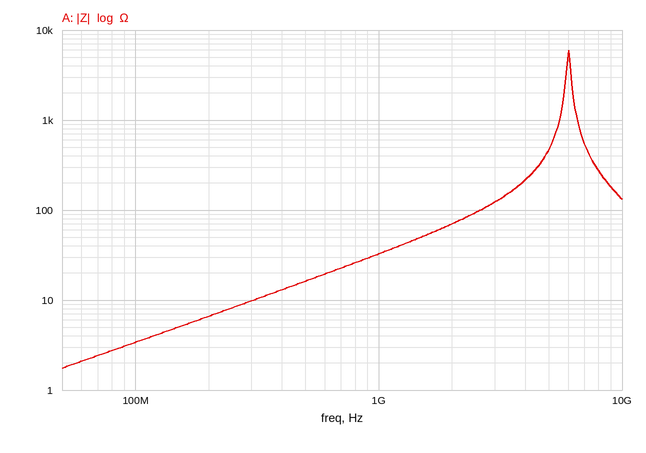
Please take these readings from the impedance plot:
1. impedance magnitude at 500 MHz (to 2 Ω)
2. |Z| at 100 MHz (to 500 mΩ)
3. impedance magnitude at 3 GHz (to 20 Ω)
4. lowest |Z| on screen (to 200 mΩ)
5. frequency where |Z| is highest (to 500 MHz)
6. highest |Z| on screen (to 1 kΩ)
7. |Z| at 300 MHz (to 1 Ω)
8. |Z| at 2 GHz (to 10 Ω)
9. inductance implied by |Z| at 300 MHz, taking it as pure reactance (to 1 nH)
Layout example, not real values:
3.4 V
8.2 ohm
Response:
16 Ω
3.5 Ω
120 Ω
1.8 Ω
6.0 GHz
6 kΩ
10 Ω
70 Ω
5 nH
